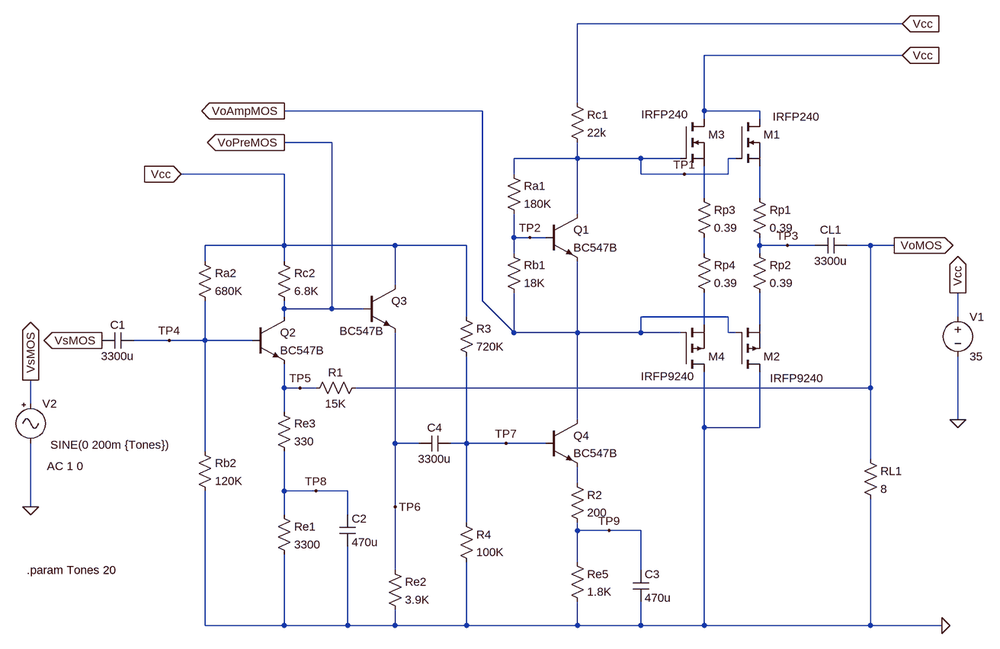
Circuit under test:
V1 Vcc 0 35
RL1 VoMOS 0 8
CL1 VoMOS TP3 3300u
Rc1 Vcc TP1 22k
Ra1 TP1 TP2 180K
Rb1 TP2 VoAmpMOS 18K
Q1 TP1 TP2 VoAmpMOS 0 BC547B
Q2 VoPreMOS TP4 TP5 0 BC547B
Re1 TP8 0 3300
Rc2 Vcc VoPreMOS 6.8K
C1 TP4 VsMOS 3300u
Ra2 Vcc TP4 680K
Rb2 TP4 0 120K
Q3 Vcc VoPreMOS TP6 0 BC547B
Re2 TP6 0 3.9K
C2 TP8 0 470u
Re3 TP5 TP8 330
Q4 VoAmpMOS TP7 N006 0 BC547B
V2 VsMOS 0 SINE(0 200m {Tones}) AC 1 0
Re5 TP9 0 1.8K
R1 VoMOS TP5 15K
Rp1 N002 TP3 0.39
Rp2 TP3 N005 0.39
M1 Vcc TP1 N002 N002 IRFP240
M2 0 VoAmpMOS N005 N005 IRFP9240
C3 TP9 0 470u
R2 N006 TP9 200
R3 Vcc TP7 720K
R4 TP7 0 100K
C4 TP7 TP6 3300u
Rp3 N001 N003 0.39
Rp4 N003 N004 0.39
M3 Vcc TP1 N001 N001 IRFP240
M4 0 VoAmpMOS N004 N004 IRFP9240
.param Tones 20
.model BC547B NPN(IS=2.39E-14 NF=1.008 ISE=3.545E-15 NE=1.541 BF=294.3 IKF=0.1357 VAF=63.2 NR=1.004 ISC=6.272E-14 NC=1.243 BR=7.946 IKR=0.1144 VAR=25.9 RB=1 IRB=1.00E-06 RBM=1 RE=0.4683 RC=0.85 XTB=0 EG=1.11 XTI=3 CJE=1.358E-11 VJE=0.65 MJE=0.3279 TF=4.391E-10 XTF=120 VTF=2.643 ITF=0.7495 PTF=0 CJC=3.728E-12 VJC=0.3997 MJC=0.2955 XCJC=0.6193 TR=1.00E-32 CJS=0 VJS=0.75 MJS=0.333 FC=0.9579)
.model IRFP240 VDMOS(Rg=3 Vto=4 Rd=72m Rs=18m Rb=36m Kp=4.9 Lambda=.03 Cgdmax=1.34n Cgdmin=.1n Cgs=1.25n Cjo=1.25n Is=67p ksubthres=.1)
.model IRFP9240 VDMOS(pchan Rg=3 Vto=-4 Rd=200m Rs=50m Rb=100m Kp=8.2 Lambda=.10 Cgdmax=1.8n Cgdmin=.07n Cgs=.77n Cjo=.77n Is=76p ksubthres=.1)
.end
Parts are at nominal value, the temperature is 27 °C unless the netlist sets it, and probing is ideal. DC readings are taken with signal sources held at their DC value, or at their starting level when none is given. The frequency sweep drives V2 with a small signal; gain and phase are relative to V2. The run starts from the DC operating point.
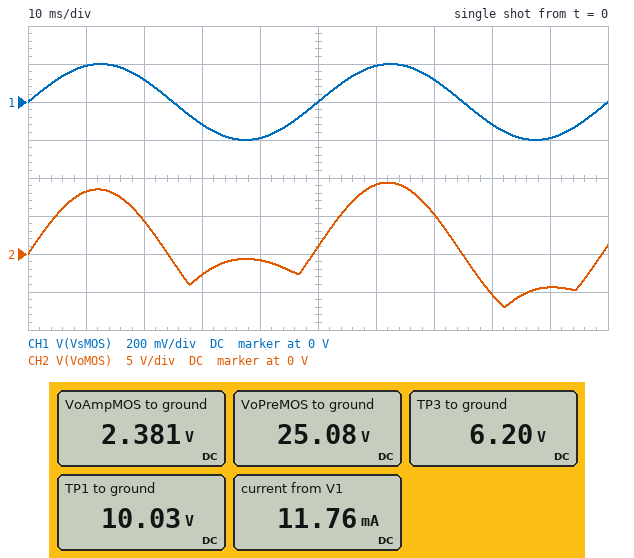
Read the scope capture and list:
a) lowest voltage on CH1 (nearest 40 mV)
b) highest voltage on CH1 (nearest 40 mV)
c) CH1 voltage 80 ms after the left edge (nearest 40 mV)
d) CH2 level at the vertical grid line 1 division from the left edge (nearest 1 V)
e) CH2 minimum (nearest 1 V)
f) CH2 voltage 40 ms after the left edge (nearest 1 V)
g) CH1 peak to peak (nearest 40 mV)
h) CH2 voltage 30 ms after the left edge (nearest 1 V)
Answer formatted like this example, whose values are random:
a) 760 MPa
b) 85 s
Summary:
a) -200 mV
b) 200 mV
c) -120 mV
d) 8 V
e) -7 V
f) -1 V
g) 400 mV
h) -3 V
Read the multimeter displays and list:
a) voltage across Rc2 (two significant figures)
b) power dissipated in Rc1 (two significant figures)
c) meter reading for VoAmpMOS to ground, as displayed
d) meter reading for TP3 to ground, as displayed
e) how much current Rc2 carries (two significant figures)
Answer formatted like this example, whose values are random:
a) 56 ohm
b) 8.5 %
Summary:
a) 9.9 V
b) 28 mW
c) 2.381 V
d) 6.20 V
e) 1.5 mA
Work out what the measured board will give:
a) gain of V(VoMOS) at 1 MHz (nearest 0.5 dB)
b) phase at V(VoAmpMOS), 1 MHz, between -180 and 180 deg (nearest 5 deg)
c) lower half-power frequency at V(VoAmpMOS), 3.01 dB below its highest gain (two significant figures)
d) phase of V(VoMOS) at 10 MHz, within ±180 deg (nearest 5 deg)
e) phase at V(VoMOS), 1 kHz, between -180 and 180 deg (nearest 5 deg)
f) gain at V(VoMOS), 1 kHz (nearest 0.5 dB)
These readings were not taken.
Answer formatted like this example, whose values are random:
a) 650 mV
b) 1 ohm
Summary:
a) 4.0 dB
b) -95 deg
c) 980 mHz
d) 170 deg
e) 0 deg
f) 25.0 dB
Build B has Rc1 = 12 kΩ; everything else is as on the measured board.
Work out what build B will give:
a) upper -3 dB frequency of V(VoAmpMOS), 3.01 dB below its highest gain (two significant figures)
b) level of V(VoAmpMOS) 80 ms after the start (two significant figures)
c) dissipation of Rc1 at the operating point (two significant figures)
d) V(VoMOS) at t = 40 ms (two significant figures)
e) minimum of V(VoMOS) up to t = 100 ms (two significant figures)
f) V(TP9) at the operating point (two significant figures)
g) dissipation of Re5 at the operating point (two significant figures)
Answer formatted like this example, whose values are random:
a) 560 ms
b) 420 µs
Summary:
a) 1.2 Hz
b) 6.6 V
c) 30 mW
d) -4.7 V
e) -8.0 V
f) 2.8 V
g) 4.5 mW
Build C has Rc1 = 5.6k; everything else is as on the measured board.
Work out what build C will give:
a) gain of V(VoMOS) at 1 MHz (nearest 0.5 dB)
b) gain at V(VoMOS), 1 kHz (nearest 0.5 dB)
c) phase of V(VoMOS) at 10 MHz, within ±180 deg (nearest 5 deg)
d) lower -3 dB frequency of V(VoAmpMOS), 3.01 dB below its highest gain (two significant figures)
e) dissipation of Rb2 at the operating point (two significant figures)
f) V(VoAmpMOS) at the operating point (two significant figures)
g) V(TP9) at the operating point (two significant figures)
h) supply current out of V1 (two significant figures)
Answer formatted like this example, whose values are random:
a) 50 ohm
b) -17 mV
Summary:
a) 26.0 dB
b) 32.5 dB
c) -165 deg
d) 680 mHz
e) 200 µW
f) 18 V
g) 2.9 V
h) 69 mA
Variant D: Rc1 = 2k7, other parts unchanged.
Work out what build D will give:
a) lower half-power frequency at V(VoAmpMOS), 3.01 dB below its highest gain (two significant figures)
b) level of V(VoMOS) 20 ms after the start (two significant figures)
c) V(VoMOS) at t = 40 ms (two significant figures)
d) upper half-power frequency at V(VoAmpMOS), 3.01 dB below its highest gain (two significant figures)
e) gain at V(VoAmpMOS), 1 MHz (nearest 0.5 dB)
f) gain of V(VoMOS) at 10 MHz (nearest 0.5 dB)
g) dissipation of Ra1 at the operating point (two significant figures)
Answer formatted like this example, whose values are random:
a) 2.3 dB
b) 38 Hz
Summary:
a) 870 mHz
b) 2.1 V
c) -7.5 V
d) 2.6 Hz
e) 28.5 dB
f) 3.0 dB
g) 300 µW
